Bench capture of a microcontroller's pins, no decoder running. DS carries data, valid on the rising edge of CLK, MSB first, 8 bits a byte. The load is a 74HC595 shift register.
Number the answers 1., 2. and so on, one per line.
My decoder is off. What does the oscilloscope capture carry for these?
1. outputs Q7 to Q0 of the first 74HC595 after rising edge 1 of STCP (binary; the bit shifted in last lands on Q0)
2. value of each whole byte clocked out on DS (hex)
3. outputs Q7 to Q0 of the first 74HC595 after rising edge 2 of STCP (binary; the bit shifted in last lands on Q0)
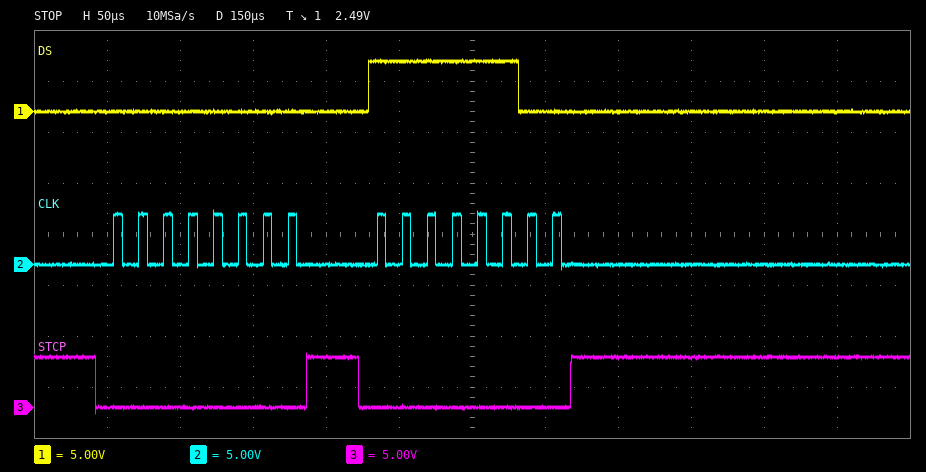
1. 00000000
2. 00 FC
3. 11111100
